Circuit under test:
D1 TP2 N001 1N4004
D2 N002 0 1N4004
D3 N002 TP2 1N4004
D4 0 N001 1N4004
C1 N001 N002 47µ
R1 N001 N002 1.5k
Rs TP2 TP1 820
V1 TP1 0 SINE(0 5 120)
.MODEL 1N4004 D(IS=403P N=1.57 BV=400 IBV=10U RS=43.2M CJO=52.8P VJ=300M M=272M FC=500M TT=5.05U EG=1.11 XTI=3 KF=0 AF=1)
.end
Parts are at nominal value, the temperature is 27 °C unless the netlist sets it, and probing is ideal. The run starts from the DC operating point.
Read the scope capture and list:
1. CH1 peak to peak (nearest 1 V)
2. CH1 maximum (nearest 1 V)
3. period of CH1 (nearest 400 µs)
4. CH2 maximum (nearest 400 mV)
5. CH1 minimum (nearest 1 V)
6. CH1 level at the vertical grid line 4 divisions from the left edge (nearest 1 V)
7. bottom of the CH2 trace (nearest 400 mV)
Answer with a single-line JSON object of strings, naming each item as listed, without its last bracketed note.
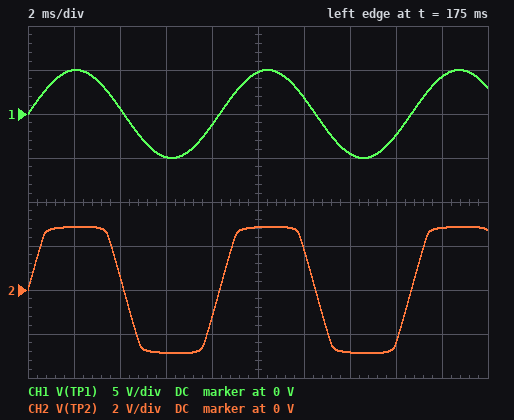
{"CH1 peak to peak": "10 V", "CH1 maximum": "5 V", "period of CH1": "8.4 ms", "CH2 maximum": "2.8 V", "CH1 minimum": "-5 V", "CH1 level at the vertical grid line 4 divisions from the left edge": "-1 V", "bottom of the CH2 trace": "-2.8 V"}
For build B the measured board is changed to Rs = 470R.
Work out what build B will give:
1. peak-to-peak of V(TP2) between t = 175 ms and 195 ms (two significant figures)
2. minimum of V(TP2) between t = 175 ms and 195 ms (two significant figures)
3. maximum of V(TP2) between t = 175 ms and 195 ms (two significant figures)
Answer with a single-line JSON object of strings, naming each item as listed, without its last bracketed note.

{"peak-to-peak of V(TP2) between t = 175 ms and 195 ms": "6.6 V", "minimum of V(TP2) between t = 175 ms and 195 ms": "-3.3 V", "maximum of V(TP2) between t = 175 ms and 195 ms": "3.3 V"}
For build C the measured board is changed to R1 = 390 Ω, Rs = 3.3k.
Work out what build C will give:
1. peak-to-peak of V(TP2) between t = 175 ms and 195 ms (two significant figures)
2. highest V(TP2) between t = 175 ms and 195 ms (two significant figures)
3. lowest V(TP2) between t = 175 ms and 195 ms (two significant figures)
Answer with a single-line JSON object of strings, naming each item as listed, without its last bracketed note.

{"peak-to-peak of V(TP2) between t = 175 ms and 195 ms": "2.9 V", "highest V(TP2) between t = 175 ms and 195 ms": "1.4 V", "lowest V(TP2) between t = 175 ms and 195 ms": "-1.4 V"}
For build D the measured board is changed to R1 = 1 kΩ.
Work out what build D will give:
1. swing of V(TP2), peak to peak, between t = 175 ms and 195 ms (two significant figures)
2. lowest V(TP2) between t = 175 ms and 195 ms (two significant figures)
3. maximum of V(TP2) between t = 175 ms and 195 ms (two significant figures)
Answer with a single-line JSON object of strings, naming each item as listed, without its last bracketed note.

{"swing of V(TP2), peak to peak, between t = 175 ms and 195 ms": "5.2 V", "lowest V(TP2) between t = 175 ms and 195 ms": "-2.6 V", "maximum of V(TP2) between t = 175 ms and 195 ms": "2.6 V"}
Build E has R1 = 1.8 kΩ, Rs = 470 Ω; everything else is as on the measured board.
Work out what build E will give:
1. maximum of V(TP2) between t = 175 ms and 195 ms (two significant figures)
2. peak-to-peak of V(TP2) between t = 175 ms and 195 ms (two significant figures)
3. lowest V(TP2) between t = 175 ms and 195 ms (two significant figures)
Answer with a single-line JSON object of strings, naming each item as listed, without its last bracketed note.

{"maximum of V(TP2) between t = 175 ms and 195 ms": "3.4 V", "peak-to-peak of V(TP2) between t = 175 ms and 195 ms": "6.9 V", "lowest V(TP2) between t = 175 ms and 195 ms": "-3.4 V"}
